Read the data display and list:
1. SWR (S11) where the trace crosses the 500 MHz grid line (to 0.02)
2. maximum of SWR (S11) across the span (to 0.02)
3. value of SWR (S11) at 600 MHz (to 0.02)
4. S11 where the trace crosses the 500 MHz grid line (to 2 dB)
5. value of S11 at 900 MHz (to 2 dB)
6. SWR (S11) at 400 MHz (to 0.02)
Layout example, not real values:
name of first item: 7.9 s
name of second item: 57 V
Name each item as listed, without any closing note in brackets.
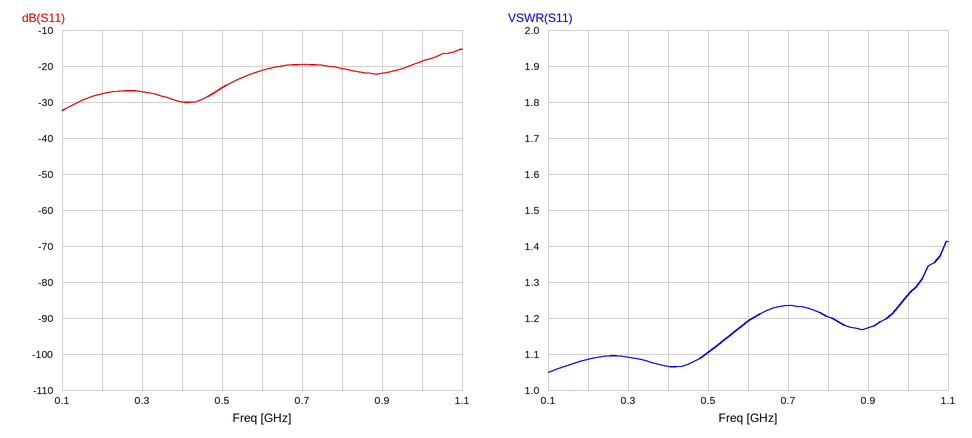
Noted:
SWR (S11) where the trace crosses the 500 MHz grid line: 1.10
maximum of SWR (S11) across the span: 1.42
value of SWR (S11) at 600 MHz: 1.20
S11 where the trace crosses the 500 MHz grid line: -26 dB
value of S11 at 900 MHz: -22 dB
SWR (S11) at 400 MHz: 1.06
